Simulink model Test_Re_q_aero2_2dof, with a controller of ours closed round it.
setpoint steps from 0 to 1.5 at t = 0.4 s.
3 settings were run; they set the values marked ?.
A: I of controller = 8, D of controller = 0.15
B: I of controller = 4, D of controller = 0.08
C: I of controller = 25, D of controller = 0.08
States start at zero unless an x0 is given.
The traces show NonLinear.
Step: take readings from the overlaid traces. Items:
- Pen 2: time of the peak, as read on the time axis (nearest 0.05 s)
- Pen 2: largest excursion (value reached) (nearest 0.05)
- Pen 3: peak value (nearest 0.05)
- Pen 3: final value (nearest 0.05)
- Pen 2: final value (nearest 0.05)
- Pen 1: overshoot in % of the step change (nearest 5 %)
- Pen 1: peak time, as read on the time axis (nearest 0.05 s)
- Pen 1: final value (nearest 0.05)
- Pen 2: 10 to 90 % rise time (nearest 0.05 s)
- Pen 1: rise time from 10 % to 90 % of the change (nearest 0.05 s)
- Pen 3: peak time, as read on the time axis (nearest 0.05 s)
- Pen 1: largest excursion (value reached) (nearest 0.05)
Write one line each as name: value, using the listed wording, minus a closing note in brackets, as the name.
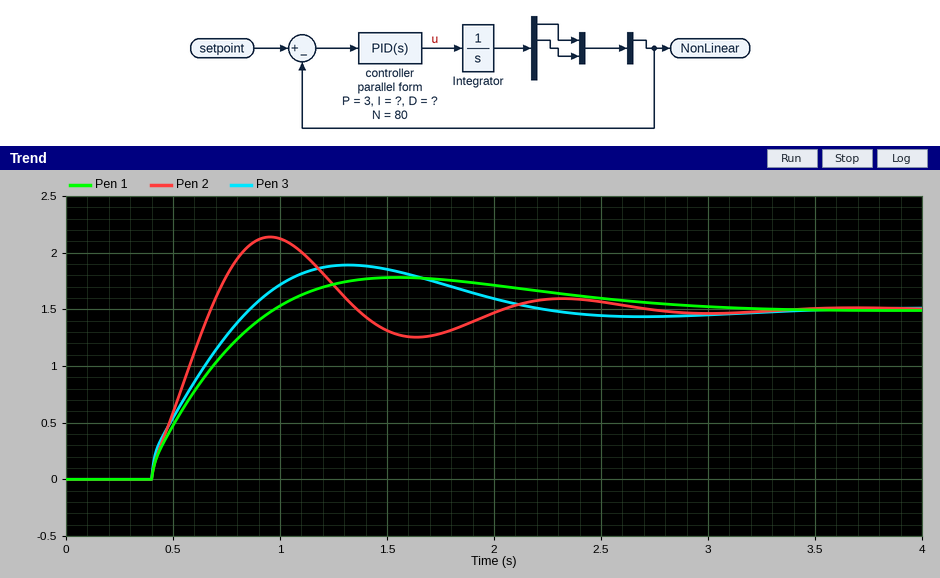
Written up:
Pen 2: time of the peak, as read on the time axis: 0.95 s
Pen 2: largest excursion (value reached): 2.15
Pen 3: peak value: 1.90
Pen 3: final value: 1.50
Pen 2: final value: 1.50
Pen 1: overshoot in % of the step change: 20 %
Pen 1: peak time, as read on the time axis: 1.55 s
Pen 1: final value: 1.50
Pen 2: 10 to 90 % rise time: 0.25 s
Pen 1: rise time from 10 % to 90 % of the change: 0.45 s
Pen 3: peak time, as read on the time axis: 1.30 s
Pen 1: largest excursion (value reached): 1.80
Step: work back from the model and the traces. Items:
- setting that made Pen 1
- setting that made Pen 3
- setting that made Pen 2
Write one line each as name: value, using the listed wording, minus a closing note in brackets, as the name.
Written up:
setting that made Pen 1: B
setting that made Pen 3: A
setting that made Pen 2: C
